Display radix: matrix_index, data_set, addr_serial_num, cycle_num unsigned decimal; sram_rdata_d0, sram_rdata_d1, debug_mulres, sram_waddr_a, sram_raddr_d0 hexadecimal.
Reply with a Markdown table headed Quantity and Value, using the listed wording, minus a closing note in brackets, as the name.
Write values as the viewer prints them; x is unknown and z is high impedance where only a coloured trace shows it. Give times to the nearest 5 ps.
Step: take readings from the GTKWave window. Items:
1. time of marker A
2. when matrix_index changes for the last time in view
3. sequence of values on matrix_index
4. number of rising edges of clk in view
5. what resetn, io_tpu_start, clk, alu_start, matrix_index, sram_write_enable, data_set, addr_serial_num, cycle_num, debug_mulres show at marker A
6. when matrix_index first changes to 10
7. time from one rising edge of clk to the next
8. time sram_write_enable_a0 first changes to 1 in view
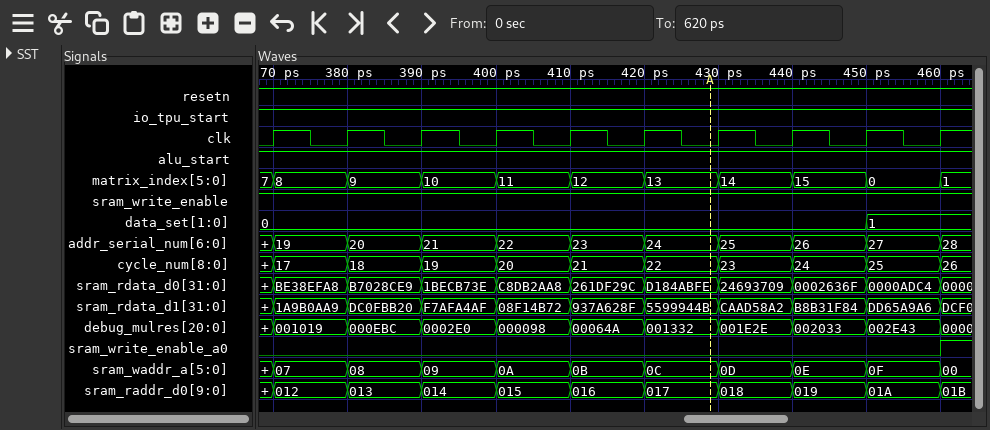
| Quantity | Value |
|---|---|
| time of marker A | 430 ps |
| when matrix_index changes for the last time in view | 460 ps |
| sequence of values on matrix_index | 7, 8, 9, 10, 11, 12, 13, 14, 15, 0, 1 |
| number of rising edges of clk in view | 10 |
| what resetn, io_tpu_start, clk, alu_start, matrix_index, sram_write_enable, data_set, addr_serial_num, cycle_num, debug_mulres show at marker A | resetn=1, io_tpu_start=1, clk=0, alu_start=1, matrix_index=13, sram_write_enable=1, data_set=0, addr_serial_num=24, cycle_num=22, debug_mulres=001332 |
| when matrix_index first changes to 10 | 390 ps |
| time from one rising edge of clk to the next | 10 ps |
| time sram_write_enable_a0 first changes to 1 in view | 460 ps |
